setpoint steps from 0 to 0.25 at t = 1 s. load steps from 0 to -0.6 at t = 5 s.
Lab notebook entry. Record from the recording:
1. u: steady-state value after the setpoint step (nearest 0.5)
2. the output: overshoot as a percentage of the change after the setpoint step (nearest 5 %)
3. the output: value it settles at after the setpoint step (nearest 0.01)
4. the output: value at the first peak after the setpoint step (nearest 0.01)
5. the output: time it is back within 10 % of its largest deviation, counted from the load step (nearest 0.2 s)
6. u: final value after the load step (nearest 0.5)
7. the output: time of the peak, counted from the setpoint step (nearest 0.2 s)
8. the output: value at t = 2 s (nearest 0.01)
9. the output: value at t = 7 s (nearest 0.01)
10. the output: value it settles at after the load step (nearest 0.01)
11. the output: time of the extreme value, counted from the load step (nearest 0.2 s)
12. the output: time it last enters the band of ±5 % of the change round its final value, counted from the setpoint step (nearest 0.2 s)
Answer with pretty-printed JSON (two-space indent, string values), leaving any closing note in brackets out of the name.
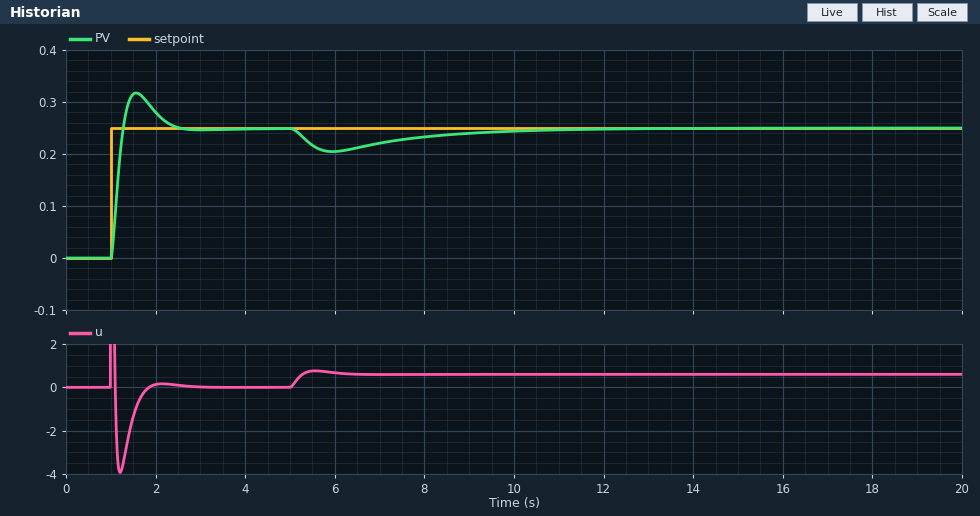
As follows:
{
  "u: steady-state value after the setpoint step": "0.0",
  "the output: overshoot as a percentage of the change after the setpoint step": "25 %",
  "the output: value it settles at after the setpoint step": "0.25",
  "the output: value at the first peak after the setpoint step": "0.32",
  "the output: time it is back within 10 % of its largest deviation, counted from the load step": "5.6 s",
  "u: final value after the load step": "0.5",
  "the output: time of the peak, counted from the setpoint step": "0.6 s",
  "the output: value at t = 2 s": "0.28",
  "the output: value at t = 7 s": "0.22",
  "the output: value it settles at after the load step": "0.25",
  "the output: time of the extreme value, counted from the load step": "1.0 s",
  "the output: time it last enters the band of ±5 % of the change round its final value, counted from the setpoint step": "1.2 s"
}
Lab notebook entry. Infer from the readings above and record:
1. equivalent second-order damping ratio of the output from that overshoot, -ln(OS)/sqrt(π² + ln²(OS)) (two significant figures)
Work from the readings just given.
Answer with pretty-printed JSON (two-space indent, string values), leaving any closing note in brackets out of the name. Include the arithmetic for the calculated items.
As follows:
{
  "equivalent second-order damping ratio of the output from that overshoot, -ln(OS)/sqrt(π² + ln²(OS))": "ln(0.25) = -1.386; 1.386 / sqrt(9.870 + 1.922) = 0.40"
}
